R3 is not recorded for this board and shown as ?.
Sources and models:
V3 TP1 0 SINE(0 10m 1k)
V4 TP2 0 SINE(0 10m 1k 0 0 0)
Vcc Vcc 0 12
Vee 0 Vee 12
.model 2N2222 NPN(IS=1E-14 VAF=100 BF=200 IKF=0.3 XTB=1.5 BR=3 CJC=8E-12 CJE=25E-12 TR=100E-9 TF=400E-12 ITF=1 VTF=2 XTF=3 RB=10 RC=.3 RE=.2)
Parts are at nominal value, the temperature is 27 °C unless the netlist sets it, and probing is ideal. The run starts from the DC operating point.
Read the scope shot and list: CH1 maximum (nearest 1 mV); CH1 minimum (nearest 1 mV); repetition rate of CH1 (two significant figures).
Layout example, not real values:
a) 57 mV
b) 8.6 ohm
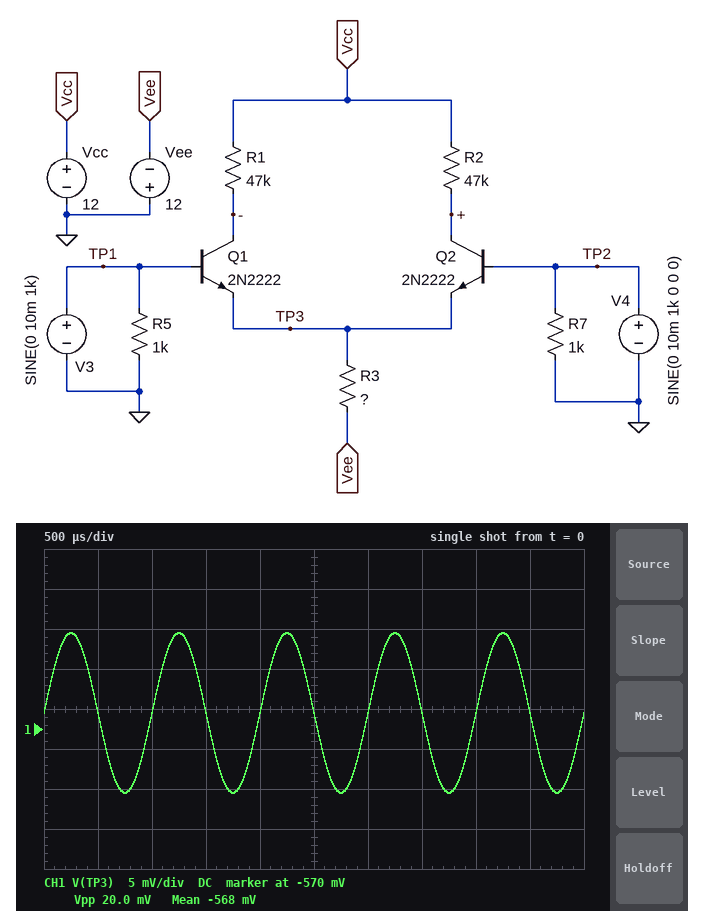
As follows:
a) -558 mV
b) -578 mV
c) 1.0 kHz
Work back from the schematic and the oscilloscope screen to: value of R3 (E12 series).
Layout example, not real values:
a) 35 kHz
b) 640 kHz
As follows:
a) 150 kΩ
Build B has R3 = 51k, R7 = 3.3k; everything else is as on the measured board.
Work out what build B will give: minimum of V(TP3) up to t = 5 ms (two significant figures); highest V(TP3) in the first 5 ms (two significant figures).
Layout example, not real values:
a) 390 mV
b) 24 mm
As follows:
a) -610 mV
b) -590 mV
